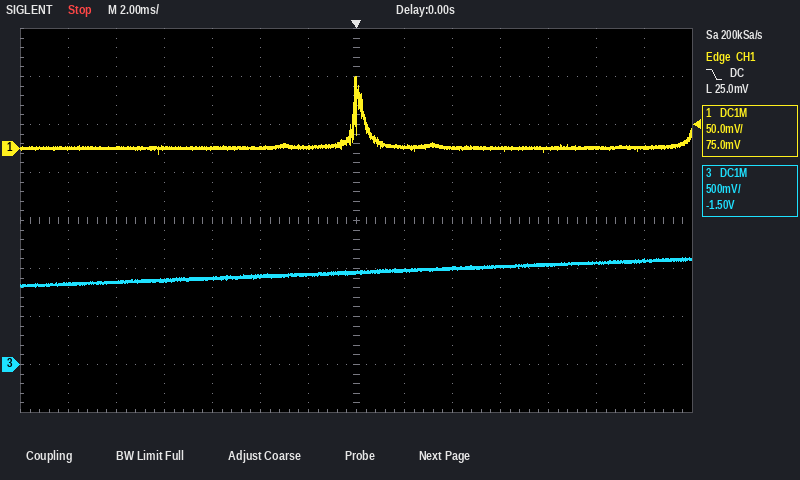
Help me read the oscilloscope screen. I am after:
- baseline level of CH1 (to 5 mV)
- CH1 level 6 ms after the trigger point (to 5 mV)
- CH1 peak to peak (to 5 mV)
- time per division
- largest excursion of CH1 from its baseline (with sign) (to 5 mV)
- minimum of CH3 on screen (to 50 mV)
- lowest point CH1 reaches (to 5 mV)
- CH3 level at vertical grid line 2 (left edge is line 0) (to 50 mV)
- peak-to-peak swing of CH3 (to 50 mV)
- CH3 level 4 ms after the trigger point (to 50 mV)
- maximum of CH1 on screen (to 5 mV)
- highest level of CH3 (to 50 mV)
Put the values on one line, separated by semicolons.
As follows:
0 mV; 0 mV; 80 mV; 2 ms; +75 mV; 800 mV; -5 mV; 850 mV; 300 mV; 1.00 V; 75 mV; 1.10 V
